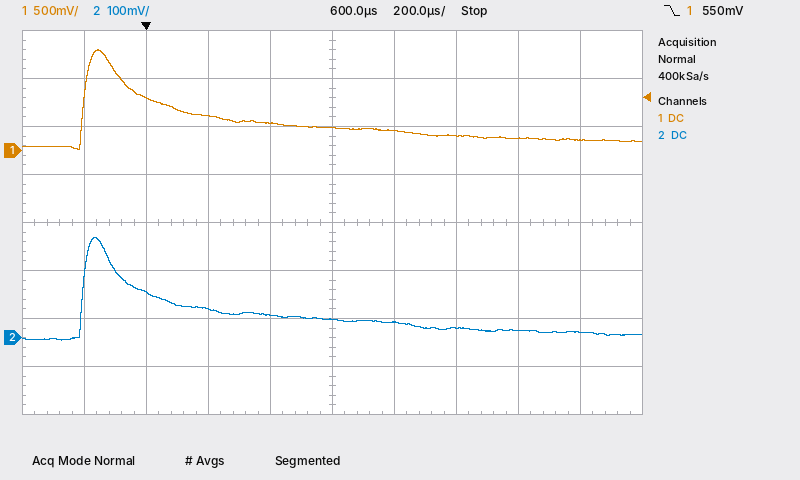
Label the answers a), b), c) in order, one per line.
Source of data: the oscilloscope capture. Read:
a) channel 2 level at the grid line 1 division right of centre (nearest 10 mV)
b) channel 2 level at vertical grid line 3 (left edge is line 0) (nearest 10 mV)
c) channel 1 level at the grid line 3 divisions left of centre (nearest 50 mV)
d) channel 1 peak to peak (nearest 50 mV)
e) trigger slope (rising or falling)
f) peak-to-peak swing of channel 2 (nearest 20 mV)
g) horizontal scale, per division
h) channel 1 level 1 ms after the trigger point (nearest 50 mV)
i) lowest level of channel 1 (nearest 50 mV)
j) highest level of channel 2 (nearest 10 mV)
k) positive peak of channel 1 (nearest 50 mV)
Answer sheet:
a) 30 mV
b) 60 mV
c) 550 mV
d) 1.05 V
e) falling
f) 220 mV
g) 200 µs
h) 150 mV
i) 0 mV
j) 210 mV
k) 1.05 V
